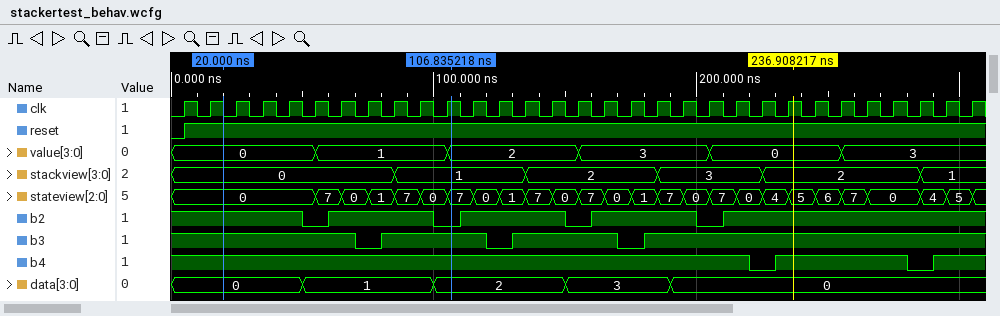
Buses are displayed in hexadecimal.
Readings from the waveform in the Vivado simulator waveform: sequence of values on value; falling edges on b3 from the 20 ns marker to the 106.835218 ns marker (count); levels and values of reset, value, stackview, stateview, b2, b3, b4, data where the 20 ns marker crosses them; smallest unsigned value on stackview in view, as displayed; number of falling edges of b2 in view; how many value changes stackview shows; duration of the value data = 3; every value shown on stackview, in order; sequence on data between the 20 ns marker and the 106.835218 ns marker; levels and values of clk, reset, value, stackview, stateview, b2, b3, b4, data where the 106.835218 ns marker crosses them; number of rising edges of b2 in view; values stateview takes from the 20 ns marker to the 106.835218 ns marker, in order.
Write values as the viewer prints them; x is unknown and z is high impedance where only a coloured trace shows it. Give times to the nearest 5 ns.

0, 1, 2, 3, 0, 3
1
reset=1, value=0, stackview=0, stateview=0, b2=1, b3=1, b4=1, data=0
0
4
5
40 ns
0, 1, 2, 3, 2, 1
0, 1, 2
clk=1, reset=1, value=2, stackview=1, stateview=7, b2=0, b3=1, b4=1, data=2
4
0, 7, 0, 1, 7, 0, 7
